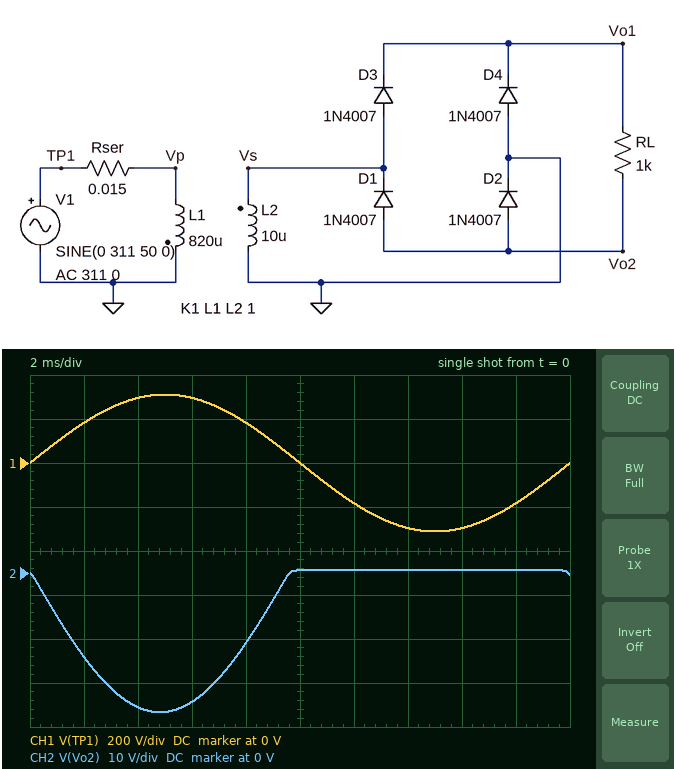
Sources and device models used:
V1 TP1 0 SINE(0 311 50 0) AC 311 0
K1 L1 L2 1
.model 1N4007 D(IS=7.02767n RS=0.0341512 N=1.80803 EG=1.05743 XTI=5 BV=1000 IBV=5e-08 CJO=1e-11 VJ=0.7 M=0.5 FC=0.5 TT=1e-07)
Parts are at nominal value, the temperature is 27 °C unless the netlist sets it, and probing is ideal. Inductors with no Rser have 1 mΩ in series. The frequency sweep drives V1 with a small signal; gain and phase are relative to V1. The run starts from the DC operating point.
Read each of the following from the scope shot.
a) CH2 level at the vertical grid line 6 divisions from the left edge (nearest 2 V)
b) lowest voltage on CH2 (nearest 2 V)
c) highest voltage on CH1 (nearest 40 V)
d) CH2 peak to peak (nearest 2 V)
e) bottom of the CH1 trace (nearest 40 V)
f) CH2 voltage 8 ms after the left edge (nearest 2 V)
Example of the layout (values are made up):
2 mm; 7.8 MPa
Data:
0 V; -32 V; 320 V; 32 V; -320 V; -16 V
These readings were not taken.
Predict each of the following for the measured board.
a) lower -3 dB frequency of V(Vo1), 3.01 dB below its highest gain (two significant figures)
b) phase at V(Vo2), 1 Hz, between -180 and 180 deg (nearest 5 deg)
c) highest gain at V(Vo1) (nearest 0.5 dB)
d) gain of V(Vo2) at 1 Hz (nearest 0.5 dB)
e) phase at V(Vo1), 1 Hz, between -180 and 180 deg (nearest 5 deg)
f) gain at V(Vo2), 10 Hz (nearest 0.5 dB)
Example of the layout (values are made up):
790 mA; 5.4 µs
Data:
3.1 Hz; -110 deg; -25.0 dB; -35.5 dB; -110 deg; -25.5 dB
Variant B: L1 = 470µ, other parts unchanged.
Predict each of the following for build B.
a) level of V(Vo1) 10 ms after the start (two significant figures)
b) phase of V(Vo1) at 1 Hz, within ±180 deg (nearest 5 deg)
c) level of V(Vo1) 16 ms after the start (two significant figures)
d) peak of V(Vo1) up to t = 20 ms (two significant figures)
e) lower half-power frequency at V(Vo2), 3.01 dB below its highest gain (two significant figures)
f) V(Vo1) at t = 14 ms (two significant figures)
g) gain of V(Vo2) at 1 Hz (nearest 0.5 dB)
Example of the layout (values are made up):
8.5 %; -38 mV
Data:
7.7 V; -100 deg; 43 V; 47 V; 5.4 Hz; 46 V; -37.5 dB
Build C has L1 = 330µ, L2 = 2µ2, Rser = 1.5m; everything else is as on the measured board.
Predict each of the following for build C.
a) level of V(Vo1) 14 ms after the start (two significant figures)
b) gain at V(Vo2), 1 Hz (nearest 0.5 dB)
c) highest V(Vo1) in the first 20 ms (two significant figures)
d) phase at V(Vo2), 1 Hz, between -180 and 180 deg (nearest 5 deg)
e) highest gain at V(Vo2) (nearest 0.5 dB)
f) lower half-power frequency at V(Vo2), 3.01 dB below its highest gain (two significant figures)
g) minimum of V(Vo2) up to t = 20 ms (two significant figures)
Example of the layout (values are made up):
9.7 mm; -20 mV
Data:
24 V; -31.5 dB; 25 V; -130 deg; -28.0 dB; 1.2 Hz; -24 V
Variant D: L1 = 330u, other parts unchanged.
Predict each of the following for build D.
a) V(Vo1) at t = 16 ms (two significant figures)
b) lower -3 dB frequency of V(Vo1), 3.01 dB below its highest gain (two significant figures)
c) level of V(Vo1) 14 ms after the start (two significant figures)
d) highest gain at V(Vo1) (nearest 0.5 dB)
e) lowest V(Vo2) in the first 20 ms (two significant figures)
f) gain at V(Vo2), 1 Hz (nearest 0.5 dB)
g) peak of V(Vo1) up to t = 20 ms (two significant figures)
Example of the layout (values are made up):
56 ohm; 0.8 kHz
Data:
51 V; 7.7 Hz; 56 V; -21.0 dB; -46 V; -39.0 dB; 57 V
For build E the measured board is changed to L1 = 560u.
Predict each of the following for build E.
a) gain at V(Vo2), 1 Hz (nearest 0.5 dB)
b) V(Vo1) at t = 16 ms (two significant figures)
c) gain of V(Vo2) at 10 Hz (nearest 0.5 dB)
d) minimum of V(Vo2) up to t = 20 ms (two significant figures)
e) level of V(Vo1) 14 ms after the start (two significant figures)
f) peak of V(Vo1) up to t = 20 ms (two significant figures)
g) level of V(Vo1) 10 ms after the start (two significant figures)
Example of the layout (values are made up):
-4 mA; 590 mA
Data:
-37.0 dB; 40 V; -24.5 dB; -37 V; 42 V; 43 V; 5.9 V
